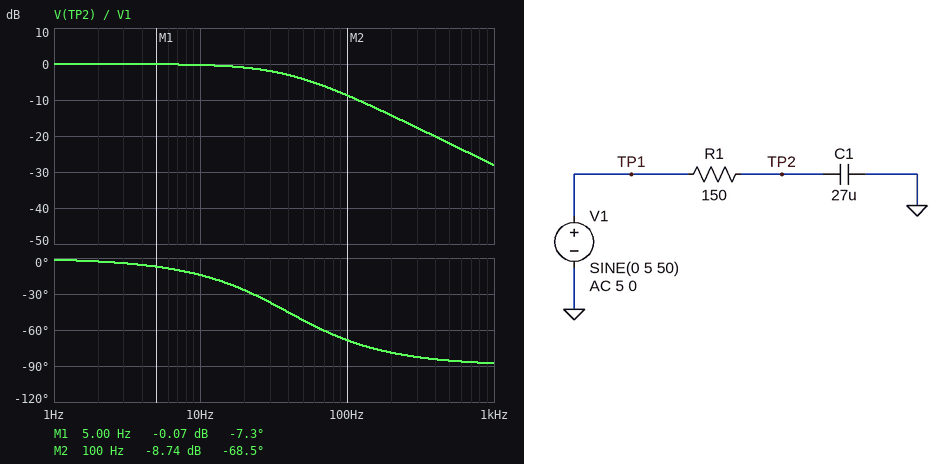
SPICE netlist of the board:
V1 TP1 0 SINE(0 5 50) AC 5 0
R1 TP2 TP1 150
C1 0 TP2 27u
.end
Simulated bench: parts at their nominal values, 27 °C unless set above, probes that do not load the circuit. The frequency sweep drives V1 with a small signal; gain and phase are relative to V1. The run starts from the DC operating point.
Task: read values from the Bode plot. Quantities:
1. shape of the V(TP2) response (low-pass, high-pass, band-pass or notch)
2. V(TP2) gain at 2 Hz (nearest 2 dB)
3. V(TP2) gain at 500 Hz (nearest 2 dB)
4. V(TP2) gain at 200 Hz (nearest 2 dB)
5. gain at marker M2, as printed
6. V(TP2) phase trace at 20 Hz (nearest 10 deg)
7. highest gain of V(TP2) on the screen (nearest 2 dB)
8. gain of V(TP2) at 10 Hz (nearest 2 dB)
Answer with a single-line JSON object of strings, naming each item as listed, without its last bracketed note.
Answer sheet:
{"shape of the V(TP2) response": "low-pass", "V(TP2) gain at 2 Hz": "0 dB", "V(TP2) gain at 500 Hz": "-22 dB", "V(TP2) gain at 200 Hz": "-14 dB", "gain at marker M2, as printed": "-8.74 dB", "V(TP2) phase trace at 20 Hz": "-30 deg", "highest gain of V(TP2) on the screen": "0 dB", "gain of V(TP2) at 10 Hz": "0 dB"}
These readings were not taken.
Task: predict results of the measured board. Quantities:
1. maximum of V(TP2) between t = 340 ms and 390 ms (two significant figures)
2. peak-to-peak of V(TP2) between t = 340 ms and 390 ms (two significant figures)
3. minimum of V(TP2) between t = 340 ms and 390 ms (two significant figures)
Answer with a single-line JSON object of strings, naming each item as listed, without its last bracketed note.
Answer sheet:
{"maximum of V(TP2) between t = 340 ms and 390 ms": "3.1 V", "peak-to-peak of V(TP2) between t = 340 ms and 390 ms": "6.2 V", "minimum of V(TP2) between t = 340 ms and 390 ms": "-3.1 V"}
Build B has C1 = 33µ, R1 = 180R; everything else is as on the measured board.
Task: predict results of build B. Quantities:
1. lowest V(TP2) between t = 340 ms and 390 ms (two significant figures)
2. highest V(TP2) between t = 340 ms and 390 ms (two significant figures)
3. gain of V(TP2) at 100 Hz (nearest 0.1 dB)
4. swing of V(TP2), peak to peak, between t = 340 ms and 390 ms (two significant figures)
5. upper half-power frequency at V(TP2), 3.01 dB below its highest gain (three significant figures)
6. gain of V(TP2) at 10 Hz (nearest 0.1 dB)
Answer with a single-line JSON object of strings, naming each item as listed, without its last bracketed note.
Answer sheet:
{"lowest V(TP2) between t = 340 ms and 390 ms": "-2.4 V", "highest V(TP2) between t = 340 ms and 390 ms": "2.4 V", "gain of V(TP2) at 100 Hz": "-11.7 dB", "swing of V(TP2), peak to peak, between t = 340 ms and 390 ms": "4.7 V", "upper half-power frequency at V(TP2), 3.01 dB below its highest gain": "26.8 Hz", "gain of V(TP2) at 10 Hz": "-0.6 dB"}
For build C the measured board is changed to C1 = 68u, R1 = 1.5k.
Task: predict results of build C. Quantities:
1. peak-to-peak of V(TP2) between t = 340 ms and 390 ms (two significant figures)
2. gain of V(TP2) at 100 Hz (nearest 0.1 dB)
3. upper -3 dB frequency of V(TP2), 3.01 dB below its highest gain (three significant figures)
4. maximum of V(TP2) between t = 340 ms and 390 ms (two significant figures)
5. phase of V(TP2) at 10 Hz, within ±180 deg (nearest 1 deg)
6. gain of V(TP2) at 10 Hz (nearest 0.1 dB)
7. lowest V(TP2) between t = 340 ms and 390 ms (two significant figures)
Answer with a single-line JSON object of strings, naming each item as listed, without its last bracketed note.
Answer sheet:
{"peak-to-peak of V(TP2) between t = 340 ms and 390 ms": "310 mV", "gain of V(TP2) at 100 Hz": "-36.1 dB", "upper -3 dB frequency of V(TP2), 3.01 dB below its highest gain": "1.56 Hz", "maximum of V(TP2) between t = 340 ms and 390 ms": "160 mV", "phase of V(TP2) at 10 Hz, within ±180 deg": "-81 deg", "gain of V(TP2) at 10 Hz": "-16.2 dB", "lowest V(TP2) between t = 340 ms and 390 ms": "-150 mV"}
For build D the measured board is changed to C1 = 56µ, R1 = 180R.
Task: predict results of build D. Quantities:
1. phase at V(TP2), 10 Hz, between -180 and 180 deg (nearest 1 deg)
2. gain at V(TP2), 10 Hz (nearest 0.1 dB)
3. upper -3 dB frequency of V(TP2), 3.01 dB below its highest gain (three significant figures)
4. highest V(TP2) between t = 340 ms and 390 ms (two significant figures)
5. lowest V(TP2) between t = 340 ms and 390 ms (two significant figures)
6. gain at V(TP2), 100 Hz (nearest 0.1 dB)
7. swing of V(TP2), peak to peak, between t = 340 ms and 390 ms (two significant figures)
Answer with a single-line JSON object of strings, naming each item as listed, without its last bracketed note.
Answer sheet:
{"phase at V(TP2), 10 Hz, between -180 and 180 deg": "-32 deg", "gain at V(TP2), 10 Hz": "-1.5 dB", "upper -3 dB frequency of V(TP2), 3.01 dB below its highest gain": "15.8 Hz", "highest V(TP2) between t = 340 ms and 390 ms": "1.5 V", "lowest V(TP2) between t = 340 ms and 390 ms": "-1.5 V", "gain at V(TP2), 100 Hz": "-16.1 dB", "swing of V(TP2), peak to peak, between t = 340 ms and 390 ms": "3.0 V"}
